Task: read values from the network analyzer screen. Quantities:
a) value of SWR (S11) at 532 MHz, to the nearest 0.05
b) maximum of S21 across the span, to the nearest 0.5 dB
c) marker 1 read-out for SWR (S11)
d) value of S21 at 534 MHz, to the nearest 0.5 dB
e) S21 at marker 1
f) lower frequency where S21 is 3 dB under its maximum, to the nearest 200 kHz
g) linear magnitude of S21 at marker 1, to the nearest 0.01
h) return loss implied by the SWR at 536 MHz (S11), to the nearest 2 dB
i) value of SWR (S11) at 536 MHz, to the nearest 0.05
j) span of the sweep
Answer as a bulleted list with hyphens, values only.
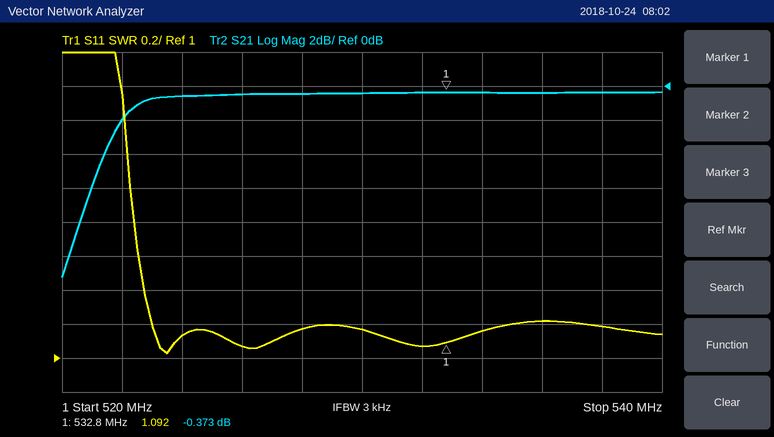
- 1.05
- -0.5 dB
- 1.092
- -0.5 dB
- -0.373 dB
- 521.6 MHz
- 0.96
- 20 dB
- 1.20
- 20 MHz
